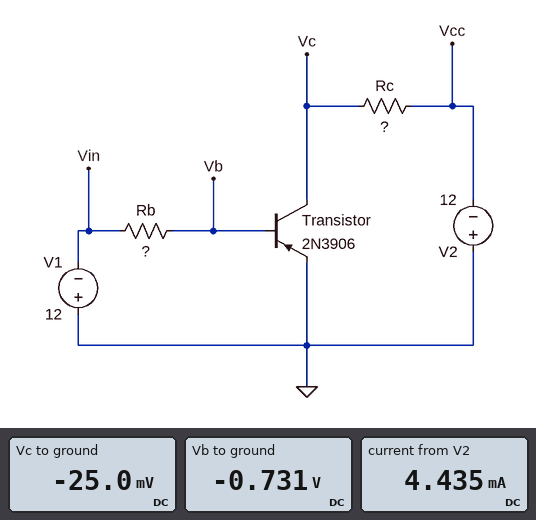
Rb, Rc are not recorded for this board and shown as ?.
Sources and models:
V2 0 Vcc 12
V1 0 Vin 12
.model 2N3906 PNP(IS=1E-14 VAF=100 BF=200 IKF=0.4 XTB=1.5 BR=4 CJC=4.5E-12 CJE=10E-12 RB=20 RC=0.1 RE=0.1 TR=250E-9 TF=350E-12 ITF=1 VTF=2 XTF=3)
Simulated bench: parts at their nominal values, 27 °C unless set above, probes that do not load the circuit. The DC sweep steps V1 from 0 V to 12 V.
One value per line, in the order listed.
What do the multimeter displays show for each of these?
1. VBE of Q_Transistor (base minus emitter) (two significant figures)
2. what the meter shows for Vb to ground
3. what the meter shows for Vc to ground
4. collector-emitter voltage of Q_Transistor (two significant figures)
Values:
-730 mV
-0.731 V
-25.0 mV
-25 mV
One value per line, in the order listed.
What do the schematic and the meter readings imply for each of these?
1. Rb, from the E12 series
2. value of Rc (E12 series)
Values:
12 kΩ
2.7 kΩ
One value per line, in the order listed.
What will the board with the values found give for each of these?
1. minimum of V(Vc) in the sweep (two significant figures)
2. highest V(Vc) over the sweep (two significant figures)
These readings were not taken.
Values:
-12 V
-25 mV
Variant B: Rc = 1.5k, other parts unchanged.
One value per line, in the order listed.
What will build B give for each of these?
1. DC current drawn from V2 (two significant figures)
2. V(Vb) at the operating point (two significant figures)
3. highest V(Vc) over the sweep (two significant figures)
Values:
8.0 mA
-740 mV
-35 mV
